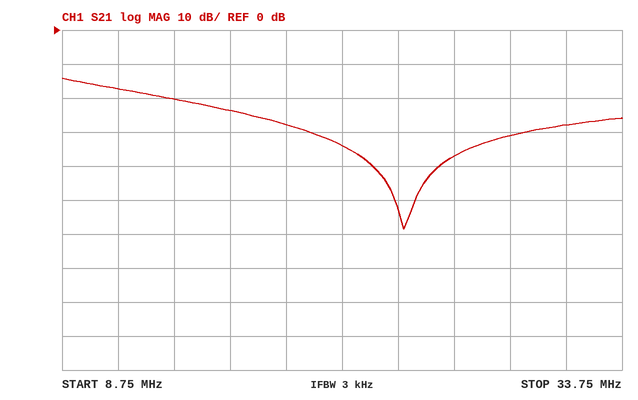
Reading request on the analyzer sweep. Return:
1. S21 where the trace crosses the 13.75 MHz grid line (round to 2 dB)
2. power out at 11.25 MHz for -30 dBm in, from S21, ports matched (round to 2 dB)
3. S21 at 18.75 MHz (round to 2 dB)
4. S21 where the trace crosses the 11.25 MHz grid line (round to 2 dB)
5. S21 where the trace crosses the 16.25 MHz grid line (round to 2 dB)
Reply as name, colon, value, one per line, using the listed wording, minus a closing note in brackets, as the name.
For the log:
S21 where the trace crosses the 13.75 MHz grid line: -20 dB
power out at 11.25 MHz for -30 dBm in, from S21, ports matched: -48 dBm
S21 at 18.75 MHz: -28 dB
S21 where the trace crosses the 11.25 MHz grid line: -18 dB
S21 where the trace crosses the 16.25 MHz grid line: -24 dB
